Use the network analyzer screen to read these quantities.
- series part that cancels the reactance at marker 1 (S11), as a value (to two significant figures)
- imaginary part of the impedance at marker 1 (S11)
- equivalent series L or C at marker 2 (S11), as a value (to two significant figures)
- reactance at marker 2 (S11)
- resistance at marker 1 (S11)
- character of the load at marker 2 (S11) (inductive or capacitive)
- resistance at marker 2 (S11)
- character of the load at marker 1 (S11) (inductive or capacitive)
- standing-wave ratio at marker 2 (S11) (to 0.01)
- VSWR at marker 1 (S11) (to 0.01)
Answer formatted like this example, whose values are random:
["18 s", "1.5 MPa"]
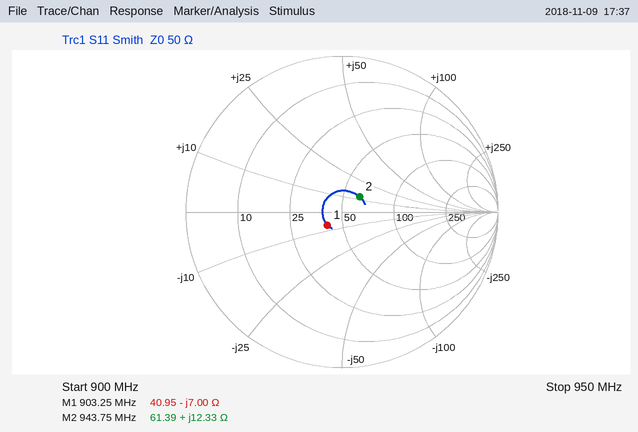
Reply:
["1.2 nH", "-7.00 Ω", "2.1 nH", "+12.33 Ω", "40.95 Ω", "inductive", "61.39 Ω", "capacitive", "1.35", "1.29"]
